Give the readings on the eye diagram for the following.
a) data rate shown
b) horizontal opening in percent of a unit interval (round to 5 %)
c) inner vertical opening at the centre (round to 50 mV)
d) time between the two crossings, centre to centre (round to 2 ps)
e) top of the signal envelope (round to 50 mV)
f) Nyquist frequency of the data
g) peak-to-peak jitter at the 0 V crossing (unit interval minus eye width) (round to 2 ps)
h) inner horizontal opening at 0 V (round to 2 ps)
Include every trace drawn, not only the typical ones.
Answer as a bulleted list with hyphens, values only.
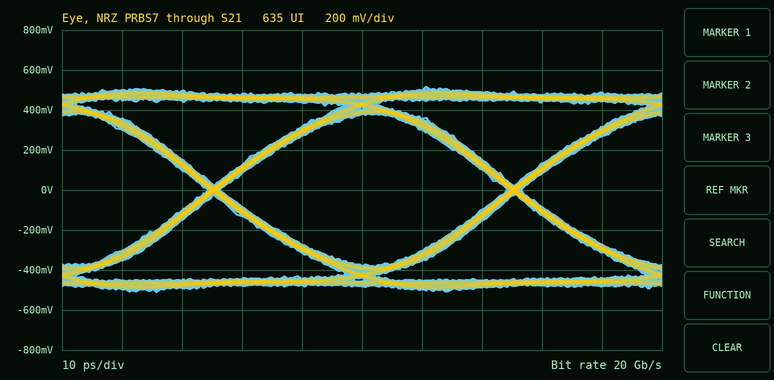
- 20 Gb/s
- 95 %
- 750 mV
- 50 ps
- 500 mV
- 10 GHz
- 2 ps
- 48 ps
